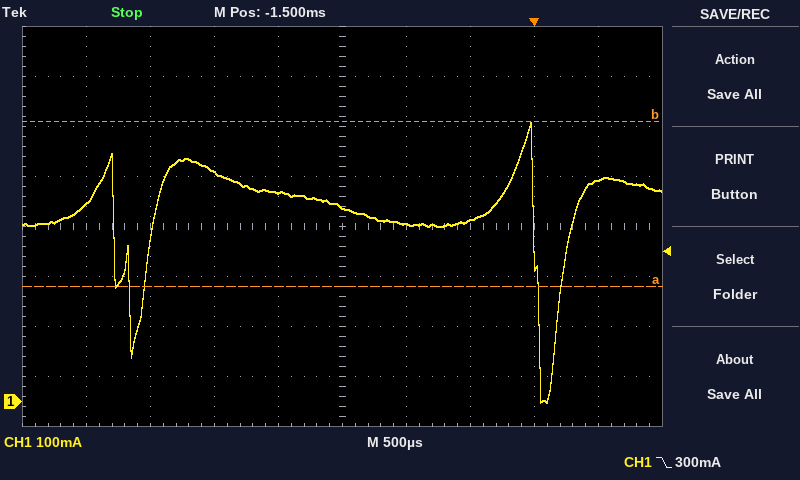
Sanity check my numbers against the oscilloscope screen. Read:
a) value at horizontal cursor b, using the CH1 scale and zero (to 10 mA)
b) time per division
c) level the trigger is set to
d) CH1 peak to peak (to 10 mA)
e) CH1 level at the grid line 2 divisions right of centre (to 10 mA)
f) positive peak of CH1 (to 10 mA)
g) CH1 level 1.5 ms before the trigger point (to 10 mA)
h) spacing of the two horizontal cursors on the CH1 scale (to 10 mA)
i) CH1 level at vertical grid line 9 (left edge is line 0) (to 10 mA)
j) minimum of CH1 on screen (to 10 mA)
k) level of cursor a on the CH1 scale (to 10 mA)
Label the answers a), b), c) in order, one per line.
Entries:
a) 560 mA
b) 500 µs
c) 300 mA
d) 560 mA
e) 360 mA
f) 560 mA
g) 390 mA
h) 330 mA
i) 440 mA
j) 0 mA
k) 230 mA
